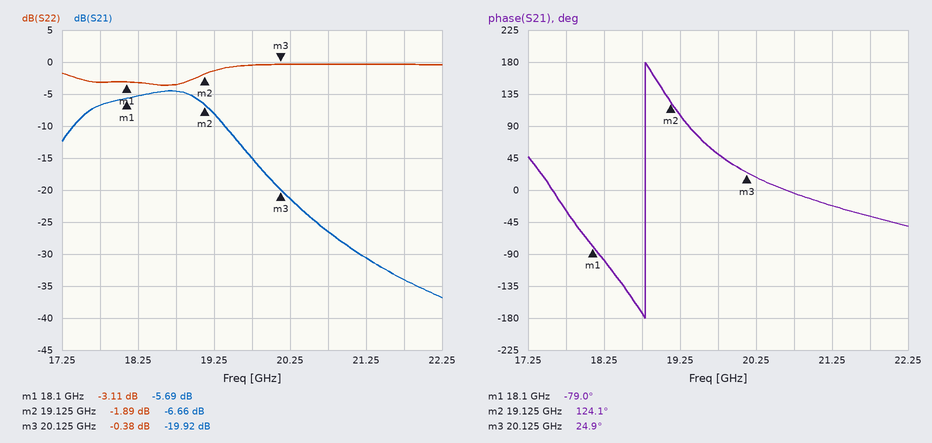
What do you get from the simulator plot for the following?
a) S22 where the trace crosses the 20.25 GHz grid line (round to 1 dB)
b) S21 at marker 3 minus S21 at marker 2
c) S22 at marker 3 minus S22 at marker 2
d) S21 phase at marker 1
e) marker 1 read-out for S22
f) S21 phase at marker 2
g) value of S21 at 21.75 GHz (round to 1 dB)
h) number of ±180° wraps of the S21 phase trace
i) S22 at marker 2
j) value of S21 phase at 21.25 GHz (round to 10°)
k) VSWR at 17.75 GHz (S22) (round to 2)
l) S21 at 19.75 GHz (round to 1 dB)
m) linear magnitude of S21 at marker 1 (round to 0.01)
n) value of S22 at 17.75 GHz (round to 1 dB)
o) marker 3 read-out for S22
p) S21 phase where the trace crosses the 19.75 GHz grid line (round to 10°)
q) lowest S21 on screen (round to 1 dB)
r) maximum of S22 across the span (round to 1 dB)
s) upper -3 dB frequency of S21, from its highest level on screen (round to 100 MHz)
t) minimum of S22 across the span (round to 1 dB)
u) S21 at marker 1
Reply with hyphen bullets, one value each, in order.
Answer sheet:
- 0 dB
- -13.26 dB
- 1.51 dB
- -79.0°
- -3.11 dB
- 124.1°
- -34 dB
- 1
- -1.89 dB
- -20°
- 6
- -15 dB
- 0.52
- -3 dB
- -0.38 dB
- 50°
- -37 dB
- 0 dB
- 19.2 GHz
- -4 dB
- -5.69 dB
